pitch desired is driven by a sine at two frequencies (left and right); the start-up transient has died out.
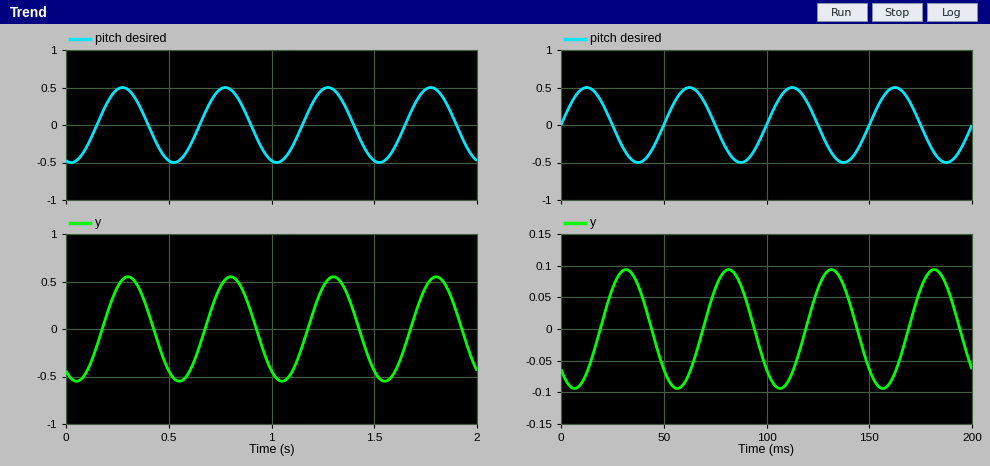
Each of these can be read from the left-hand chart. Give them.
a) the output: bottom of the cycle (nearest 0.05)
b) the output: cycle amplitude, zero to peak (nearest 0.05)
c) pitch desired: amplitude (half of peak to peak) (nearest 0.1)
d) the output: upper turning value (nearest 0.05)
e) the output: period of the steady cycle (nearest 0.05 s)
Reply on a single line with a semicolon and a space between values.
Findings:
-0.55; 0.55; 0.5; 0.55; 0.50 s
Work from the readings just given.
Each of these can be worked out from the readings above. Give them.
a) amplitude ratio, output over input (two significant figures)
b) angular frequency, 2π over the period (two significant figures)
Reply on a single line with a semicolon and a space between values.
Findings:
1.1; 13 rad/s
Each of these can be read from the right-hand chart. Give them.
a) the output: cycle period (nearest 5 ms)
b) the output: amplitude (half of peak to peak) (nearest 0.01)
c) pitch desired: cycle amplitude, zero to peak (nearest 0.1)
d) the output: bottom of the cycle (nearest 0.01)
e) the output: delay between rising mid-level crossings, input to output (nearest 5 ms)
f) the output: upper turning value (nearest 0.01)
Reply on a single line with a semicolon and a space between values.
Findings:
50 ms; 0.09; 0.5; -0.09; 20 ms; 0.09
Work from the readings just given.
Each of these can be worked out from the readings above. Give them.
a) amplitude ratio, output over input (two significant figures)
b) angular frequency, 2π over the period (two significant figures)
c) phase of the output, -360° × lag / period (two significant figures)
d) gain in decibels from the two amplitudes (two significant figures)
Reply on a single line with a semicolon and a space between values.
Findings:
0.18; 0.13 rad/ms; -140°; -15 dB
